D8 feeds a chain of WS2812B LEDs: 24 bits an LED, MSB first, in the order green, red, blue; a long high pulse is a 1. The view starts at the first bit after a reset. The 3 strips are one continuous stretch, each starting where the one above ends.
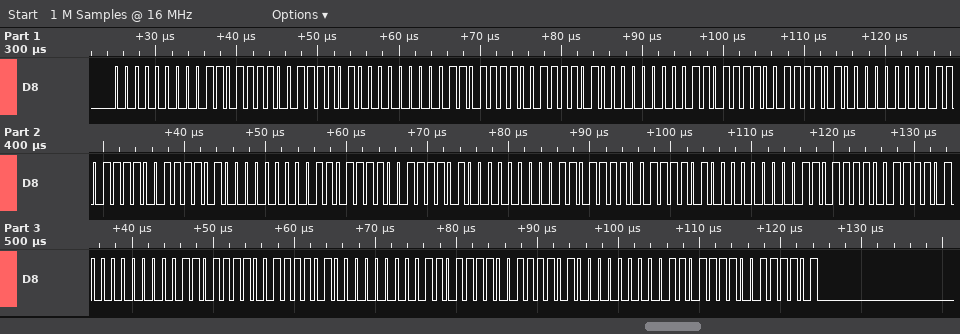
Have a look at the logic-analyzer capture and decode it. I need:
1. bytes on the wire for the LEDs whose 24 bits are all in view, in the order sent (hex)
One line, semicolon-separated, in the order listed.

00 6F 3D 00 6F 3D 00 6F 3D 00 6F 3D 00 6F 3D 00 6F 3D 00 6F 3D 00 6F 3D 00 6F 3D 00 6F 3D
